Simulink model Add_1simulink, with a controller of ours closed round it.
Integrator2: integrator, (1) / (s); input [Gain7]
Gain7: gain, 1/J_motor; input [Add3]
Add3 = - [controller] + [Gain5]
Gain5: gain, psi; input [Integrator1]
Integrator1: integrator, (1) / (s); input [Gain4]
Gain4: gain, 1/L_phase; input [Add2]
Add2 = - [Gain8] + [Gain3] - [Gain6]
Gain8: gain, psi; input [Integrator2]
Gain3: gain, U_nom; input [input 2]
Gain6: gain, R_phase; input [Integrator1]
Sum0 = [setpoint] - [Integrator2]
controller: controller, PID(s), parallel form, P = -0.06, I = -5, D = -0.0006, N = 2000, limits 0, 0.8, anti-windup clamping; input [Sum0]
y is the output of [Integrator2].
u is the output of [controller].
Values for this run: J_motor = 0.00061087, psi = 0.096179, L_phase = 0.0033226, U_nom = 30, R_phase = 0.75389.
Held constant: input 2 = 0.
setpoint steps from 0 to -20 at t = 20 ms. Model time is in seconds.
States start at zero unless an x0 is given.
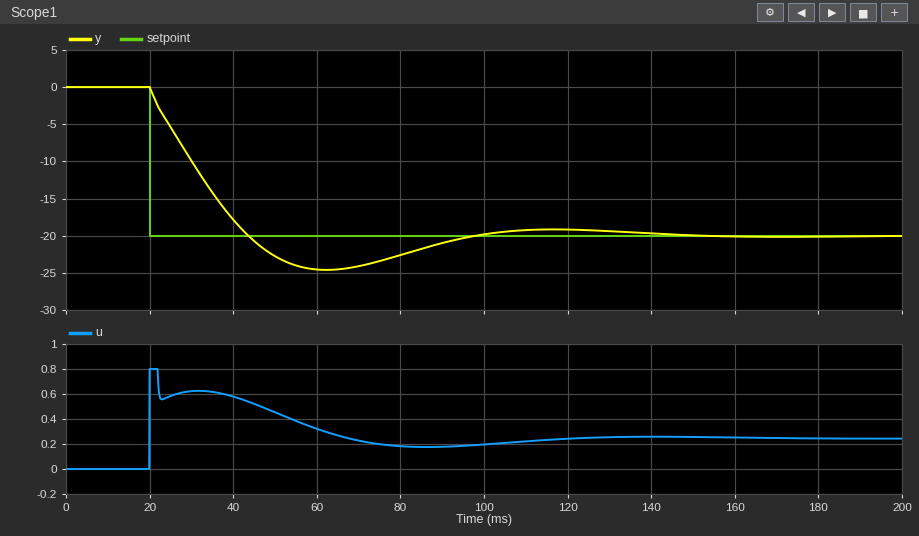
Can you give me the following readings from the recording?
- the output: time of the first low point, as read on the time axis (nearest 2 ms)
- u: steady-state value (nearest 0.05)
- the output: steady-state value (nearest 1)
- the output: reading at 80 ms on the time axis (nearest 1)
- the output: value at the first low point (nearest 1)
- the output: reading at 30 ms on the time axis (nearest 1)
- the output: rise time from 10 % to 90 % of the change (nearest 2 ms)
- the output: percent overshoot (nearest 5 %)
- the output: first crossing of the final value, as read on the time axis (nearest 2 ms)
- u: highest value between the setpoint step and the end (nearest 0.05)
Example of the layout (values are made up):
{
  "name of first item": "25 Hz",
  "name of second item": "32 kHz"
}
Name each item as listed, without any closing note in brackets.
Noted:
{
  "the output: time of the first low point, as read on the time axis": "62 ms",
  "u: steady-state value": "0.25",
  "the output: steady-state value": "-20",
  "the output: reading at 80 ms on the time axis": "-23",
  "the output: value at the first low point": "-25",
  "the output: reading at 30 ms on the time axis": "-10",
  "the output: rise time from 10 % to 90 % of the change": "18 ms",
  "the output: percent overshoot": "25 %",
  "the output: first crossing of the final value, as read on the time axis": "44 ms",
  "u: highest value between the setpoint step and the end": "0.80"
}
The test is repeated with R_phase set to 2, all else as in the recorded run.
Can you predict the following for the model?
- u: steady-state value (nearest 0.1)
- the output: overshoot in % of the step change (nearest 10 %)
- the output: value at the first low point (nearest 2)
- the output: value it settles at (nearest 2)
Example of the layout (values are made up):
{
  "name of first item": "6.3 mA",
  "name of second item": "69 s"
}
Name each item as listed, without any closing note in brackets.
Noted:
{
  "u: steady-state value": "0.1",
  "the output: overshoot in % of the step change": "30 %",
  "the output: value at the first low point": "-26",
  "the output: value it settles at": "-20"
}
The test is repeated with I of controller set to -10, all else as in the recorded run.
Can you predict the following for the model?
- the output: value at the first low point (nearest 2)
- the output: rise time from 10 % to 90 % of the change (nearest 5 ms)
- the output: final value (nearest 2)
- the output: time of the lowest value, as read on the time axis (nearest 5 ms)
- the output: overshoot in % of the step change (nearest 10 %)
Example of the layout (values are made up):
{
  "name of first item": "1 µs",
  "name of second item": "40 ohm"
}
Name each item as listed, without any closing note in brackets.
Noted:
{
  "the output: value at the first low point": "-26",
  "the output: rise time from 10 % to 90 % of the change": "15 ms",
  "the output: final value": "-20",
  "the output: time of the lowest value, as read on the time axis": "50 ms",
  "the output: overshoot in % of the step change": "30 %"
}
